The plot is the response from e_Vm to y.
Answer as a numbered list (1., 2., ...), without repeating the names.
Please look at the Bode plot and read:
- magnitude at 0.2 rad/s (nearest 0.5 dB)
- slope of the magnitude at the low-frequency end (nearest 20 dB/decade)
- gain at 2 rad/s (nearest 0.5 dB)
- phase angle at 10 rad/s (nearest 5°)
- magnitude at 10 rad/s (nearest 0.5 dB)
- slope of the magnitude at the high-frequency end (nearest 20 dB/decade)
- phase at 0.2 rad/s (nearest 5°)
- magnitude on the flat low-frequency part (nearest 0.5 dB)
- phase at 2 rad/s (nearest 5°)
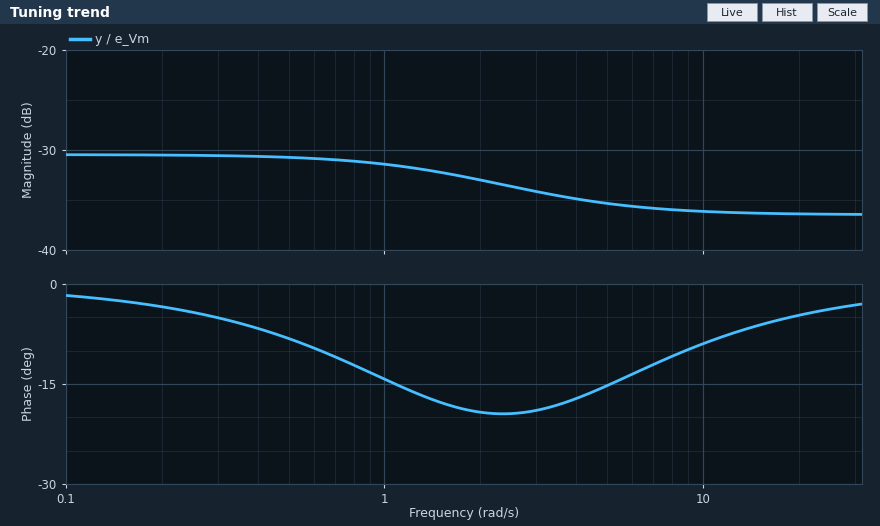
1. -30.5 dB
2. 0 dB/decade
3. -33.0 dB
4. -10°
5. -36.0 dB
6. 0 dB/decade
7. -5°
8. -30.5 dB
9. -20°
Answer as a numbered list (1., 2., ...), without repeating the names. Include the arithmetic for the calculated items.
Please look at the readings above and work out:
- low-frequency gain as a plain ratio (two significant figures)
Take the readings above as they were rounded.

1. 10^(-30.5 / 20) = 0.030
